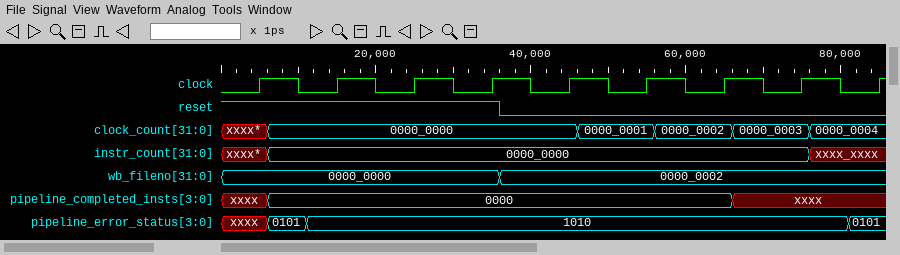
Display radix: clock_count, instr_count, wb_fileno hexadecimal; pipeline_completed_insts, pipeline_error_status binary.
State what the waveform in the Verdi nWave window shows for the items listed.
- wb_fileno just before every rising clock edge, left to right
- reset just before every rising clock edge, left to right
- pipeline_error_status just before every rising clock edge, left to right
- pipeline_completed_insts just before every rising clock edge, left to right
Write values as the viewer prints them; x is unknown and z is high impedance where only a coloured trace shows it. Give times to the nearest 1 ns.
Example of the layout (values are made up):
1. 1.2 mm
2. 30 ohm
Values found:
1. 0000_0000, 0000_0000, 0000_0000, 0000_0000, 0000_0002, 0000_0002, 0000_0002, 0000_0002, 0000_0002
2. 1 1 1 1 0 0 0 0 0
3. xxxx, 1010, 1010, 1010, 1010, 1010, 1010, 1010, 0101
4. xxxx, 0000, 0000, 0000, 0000, 0000, 0000, xxxx, xxxx
